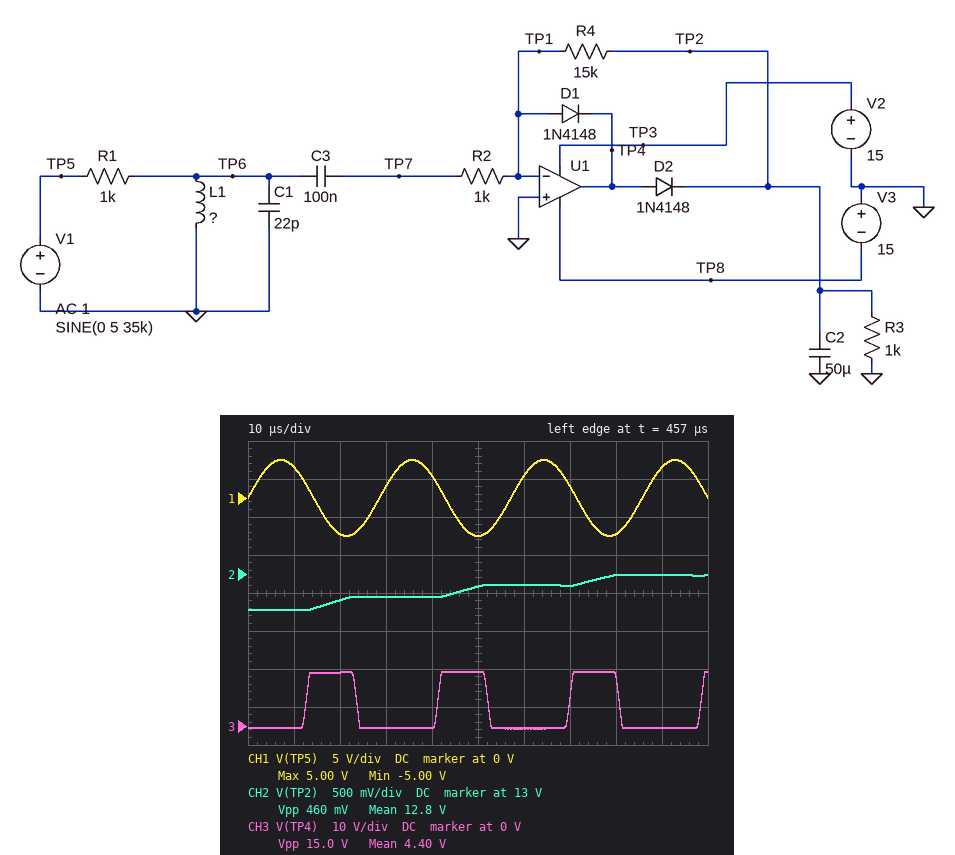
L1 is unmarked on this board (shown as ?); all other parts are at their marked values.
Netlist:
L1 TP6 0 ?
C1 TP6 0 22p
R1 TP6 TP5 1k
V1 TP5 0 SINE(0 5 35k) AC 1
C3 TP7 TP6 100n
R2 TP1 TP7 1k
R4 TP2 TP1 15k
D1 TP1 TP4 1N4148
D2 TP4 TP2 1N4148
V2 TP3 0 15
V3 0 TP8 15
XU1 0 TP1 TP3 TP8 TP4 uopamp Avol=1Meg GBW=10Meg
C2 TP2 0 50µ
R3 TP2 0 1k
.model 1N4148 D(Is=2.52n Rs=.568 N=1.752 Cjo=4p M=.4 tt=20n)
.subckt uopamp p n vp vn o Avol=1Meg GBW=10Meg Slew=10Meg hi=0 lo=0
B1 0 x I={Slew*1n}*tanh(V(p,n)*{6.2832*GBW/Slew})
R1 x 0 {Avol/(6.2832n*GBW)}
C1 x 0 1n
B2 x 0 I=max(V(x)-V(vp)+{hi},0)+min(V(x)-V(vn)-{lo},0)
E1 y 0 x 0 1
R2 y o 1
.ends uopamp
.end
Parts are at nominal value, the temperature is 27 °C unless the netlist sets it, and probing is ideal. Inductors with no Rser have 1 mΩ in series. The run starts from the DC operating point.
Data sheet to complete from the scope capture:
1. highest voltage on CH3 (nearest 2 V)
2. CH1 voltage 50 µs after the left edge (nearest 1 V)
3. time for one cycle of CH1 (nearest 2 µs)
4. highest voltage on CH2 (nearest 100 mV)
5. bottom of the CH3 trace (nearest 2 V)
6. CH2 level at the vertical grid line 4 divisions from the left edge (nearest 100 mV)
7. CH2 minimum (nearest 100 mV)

14 V
-5 V
28 µs
13.0 V
0 V
12.7 V
12.5 V
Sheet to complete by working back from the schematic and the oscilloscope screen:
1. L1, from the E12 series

2.2 mH
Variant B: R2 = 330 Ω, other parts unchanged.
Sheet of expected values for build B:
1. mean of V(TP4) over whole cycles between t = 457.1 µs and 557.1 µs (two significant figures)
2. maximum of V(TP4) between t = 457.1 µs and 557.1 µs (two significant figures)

6.7 V
15 V
